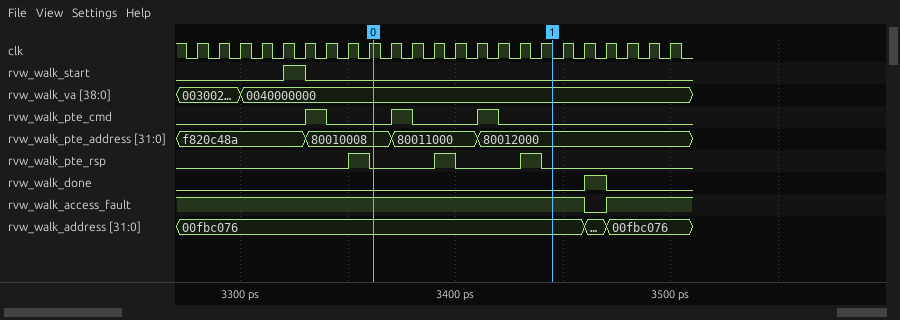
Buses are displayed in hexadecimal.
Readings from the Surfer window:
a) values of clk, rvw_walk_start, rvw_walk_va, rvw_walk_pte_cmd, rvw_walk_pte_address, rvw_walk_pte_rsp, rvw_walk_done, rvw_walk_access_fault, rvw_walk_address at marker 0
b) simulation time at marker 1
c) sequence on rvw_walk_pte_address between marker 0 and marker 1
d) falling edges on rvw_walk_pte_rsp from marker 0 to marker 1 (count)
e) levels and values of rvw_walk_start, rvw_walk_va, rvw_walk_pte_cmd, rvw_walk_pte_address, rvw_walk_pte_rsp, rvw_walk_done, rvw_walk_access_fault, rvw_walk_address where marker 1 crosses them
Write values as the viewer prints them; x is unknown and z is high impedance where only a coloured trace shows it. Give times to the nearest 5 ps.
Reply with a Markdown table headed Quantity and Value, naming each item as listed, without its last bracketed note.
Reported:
| Quantity | Value |
|---|---|
| values of clk, rvw_walk_start, rvw_walk_va, rvw_walk_pte_cmd, rvw_walk_pte_address, rvw_walk_pte_rsp, rvw_walk_done, rvw_walk_access_fault, rvw_walk_address at marker 0 | clk=1, rvw_walk_start=0, rvw_walk_va=0040000000, rvw_walk_pte_cmd=0, rvw_walk_pte_address=80010008, rvw_walk_pte_rsp=0, rvw_walk_done=0, rvw_walk_access_fault=1, rvw_walk_address=00fbc076 |
| simulation time at marker 1 | 3445 ps |
| sequence on rvw_walk_pte_address between marker 0 and marker 1 | 80010008, 80011000, 80012000 |
| falling edges on rvw_walk_pte_rsp from marker 0 to marker 1 | 2 |
| levels and values of rvw_walk_start, rvw_walk_va, rvw_walk_pte_cmd, rvw_walk_pte_address, rvw_walk_pte_rsp, rvw_walk_done, rvw_walk_access_fault, rvw_walk_address where marker 1 crosses them | rvw_walk_start=0, rvw_walk_va=0040000000, rvw_walk_pte_cmd=0, rvw_walk_pte_address=80012000, rvw_walk_pte_rsp=0, rvw_walk_done=0, rvw_walk_access_fault=1, rvw_walk_address=00fbc076 |
